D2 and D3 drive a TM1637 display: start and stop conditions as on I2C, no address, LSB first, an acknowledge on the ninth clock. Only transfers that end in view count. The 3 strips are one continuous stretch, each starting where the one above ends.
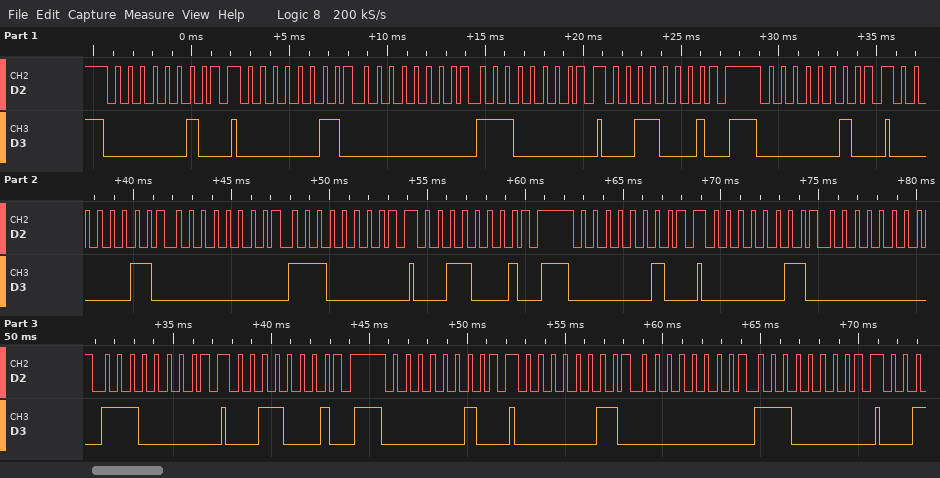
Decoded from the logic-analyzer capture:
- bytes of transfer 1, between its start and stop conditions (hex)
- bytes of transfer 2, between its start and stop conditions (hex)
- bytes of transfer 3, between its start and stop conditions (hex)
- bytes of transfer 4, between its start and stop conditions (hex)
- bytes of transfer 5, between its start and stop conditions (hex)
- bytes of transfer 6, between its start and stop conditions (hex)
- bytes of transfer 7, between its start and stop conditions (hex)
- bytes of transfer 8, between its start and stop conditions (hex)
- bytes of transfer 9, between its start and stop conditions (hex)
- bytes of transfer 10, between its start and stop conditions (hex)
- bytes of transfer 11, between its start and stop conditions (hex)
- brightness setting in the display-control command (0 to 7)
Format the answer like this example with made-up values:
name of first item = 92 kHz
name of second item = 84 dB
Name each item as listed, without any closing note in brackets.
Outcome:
bytes of transfer 1, between its start and stop conditions = 40
bytes of transfer 2, between its start and stop conditions = C0 00 07
bytes of transfer 3, between its start and stop conditions = 8C
bytes of transfer 4, between its start and stop conditions = 40
bytes of transfer 5, between its start and stop conditions = C0 00 07
bytes of transfer 6, between its start and stop conditions = 8C
bytes of transfer 7, between its start and stop conditions = 40
bytes of transfer 8, between its start and stop conditions = C0 00 07
bytes of transfer 9, between its start and stop conditions = 8C
bytes of transfer 10, between its start and stop conditions = 40
bytes of transfer 11, between its start and stop conditions = C0 00 07
brightness setting in the display-control command = 4
